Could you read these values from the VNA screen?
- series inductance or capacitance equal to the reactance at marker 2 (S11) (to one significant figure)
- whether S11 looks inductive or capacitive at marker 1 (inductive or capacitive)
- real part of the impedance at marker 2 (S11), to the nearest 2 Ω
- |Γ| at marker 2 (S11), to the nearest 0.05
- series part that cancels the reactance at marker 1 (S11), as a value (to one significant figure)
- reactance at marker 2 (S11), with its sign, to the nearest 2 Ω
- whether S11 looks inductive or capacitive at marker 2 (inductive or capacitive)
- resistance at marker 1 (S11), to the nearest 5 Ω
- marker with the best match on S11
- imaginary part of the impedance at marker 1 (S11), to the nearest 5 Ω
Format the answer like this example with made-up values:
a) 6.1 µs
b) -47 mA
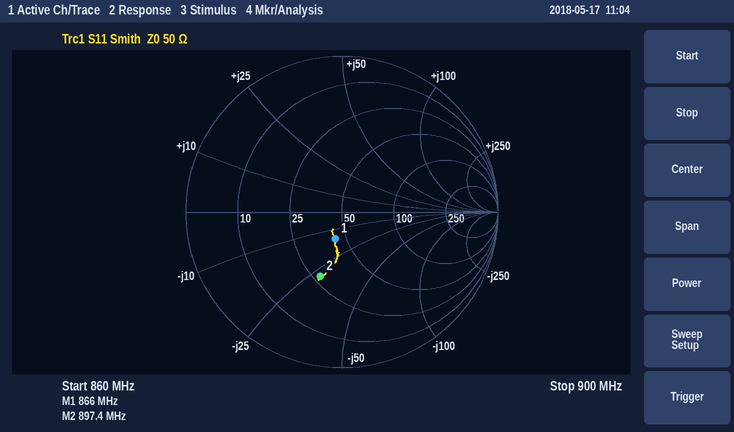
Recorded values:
a) 6 pF
b) capacitive
c) 28 Ω
d) 0.45
e) 3 nH
f) -28 Ω
g) capacitive
h) 45 Ω
i) marker 1
j) -15 Ω
